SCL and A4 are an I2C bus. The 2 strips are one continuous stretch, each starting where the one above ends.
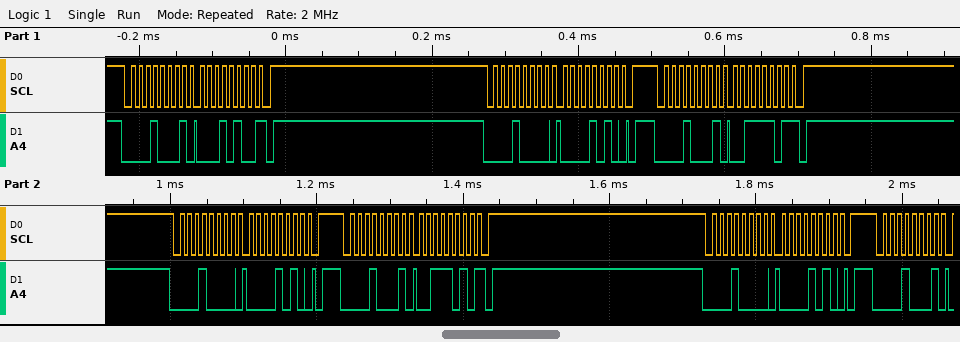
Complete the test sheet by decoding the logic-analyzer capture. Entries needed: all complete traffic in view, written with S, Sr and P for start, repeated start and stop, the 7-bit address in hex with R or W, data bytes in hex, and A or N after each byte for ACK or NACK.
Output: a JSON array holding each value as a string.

["S 08R A 14 N P S 08W A 0A A P S 08R A 3D N P S 08W A 0A A P S 08R A 3A N P S 08W A 0A A P S 08R A"]
